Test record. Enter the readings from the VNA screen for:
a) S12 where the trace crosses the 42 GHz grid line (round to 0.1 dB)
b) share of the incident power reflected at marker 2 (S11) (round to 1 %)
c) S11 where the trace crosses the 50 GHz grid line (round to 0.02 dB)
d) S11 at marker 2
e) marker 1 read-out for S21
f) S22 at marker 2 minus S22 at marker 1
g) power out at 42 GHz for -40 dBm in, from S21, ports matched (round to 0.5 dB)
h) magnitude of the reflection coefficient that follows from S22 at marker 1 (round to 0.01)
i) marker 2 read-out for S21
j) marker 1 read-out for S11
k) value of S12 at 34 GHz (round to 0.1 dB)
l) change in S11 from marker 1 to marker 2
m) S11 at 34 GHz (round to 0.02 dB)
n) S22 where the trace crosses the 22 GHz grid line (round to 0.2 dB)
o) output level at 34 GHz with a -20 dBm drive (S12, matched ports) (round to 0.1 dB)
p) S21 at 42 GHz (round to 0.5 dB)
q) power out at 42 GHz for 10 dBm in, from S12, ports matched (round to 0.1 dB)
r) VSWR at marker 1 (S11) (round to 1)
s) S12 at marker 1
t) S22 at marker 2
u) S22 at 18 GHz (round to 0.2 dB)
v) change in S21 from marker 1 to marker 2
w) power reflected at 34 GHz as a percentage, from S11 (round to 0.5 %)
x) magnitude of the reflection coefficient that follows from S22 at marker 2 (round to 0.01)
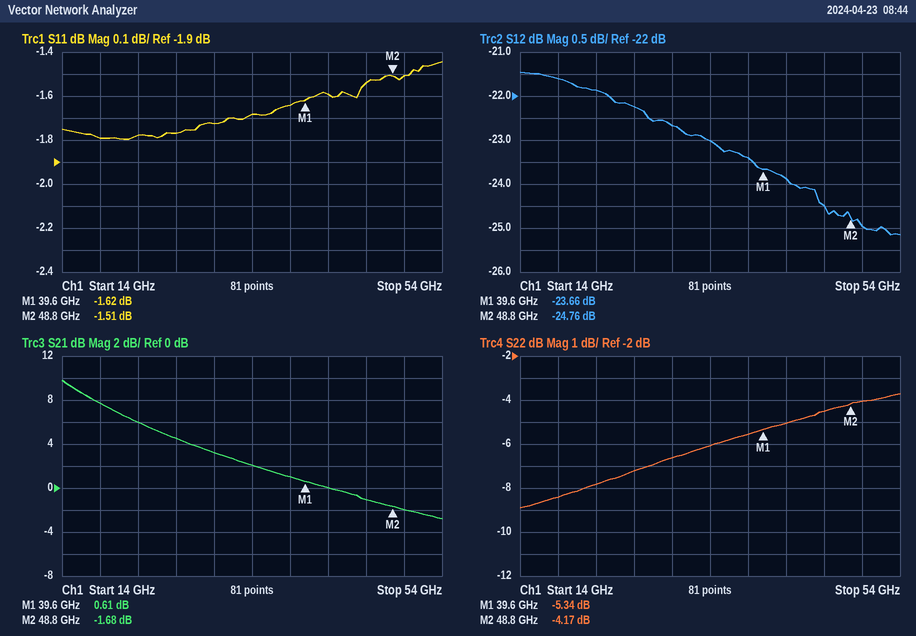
-23.9 dB
71 %
-1.50 dB
-1.51 dB
0.61 dB
1.17 dB
-40.0 dBm
0.54
-1.68 dB
-1.62 dB
-23.0 dB
0.11 dB
-1.68 dB
-7.8 dB
-43.0 dBm
0.0 dB
-13.9 dBm
11
-23.66 dB
-4.17 dB
-8.4 dB
-2.29 dB
68.0 %
0.62
